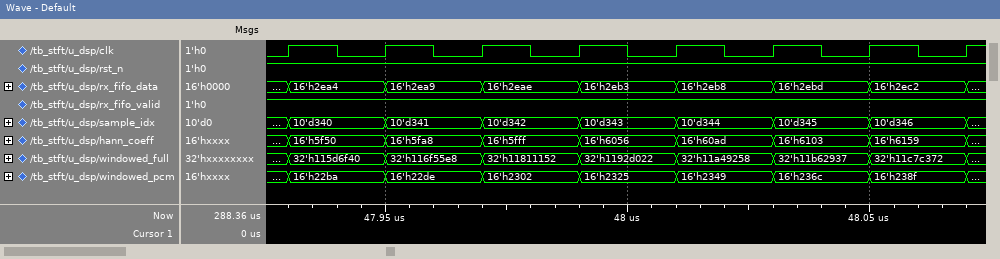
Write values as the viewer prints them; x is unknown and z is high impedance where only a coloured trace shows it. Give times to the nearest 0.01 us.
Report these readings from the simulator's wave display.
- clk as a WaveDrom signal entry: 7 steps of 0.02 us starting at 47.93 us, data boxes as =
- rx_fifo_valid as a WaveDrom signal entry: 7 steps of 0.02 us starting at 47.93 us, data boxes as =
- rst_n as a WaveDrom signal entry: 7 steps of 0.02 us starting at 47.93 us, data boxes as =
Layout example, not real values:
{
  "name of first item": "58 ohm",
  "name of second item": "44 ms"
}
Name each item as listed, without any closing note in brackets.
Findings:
{
  "clk as a WaveDrom signal entry: 7 steps of 0.02 us starting at 47.93 us, data boxes as =": "{name: 'clk', wave: 'p......'}",
  "rx_fifo_valid as a WaveDrom signal entry: 7 steps of 0.02 us starting at 47.93 us, data boxes as =": "{name: 'rx_fifo_valid', wave: '1......'}",
  "rst_n as a WaveDrom signal entry: 7 steps of 0.02 us starting at 47.93 us, data boxes as =": "{name: 'rst_n', wave: '1......'}"
}
